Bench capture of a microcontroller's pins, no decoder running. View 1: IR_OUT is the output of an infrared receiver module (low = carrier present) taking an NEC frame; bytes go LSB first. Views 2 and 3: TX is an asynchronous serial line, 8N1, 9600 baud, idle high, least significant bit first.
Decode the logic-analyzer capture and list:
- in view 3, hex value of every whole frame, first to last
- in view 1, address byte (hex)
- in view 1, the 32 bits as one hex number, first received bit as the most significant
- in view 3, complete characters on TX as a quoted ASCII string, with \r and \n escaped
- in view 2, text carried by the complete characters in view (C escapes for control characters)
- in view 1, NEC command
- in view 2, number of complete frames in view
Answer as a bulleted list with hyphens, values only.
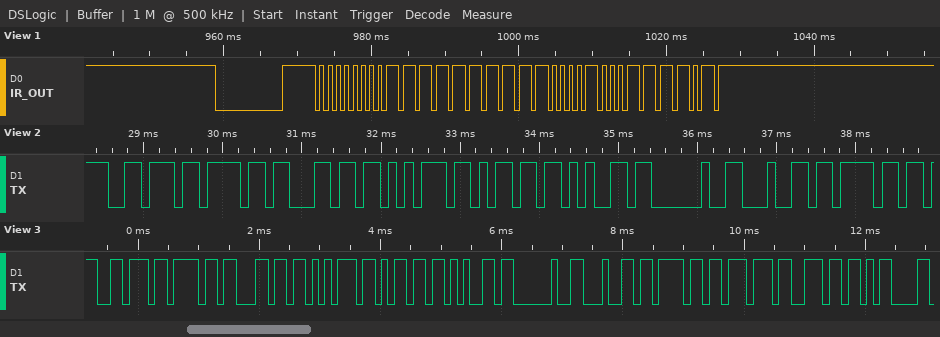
- 0x76 0x6F 0x6C 0x75 0x6D 0x65 0x20 0x64 0x6F 0x77 0x6E 0x0D
- 0x00
- 0x00FFC23D
- "volume down\r"
- "volume do"
- 0x43
- 9
